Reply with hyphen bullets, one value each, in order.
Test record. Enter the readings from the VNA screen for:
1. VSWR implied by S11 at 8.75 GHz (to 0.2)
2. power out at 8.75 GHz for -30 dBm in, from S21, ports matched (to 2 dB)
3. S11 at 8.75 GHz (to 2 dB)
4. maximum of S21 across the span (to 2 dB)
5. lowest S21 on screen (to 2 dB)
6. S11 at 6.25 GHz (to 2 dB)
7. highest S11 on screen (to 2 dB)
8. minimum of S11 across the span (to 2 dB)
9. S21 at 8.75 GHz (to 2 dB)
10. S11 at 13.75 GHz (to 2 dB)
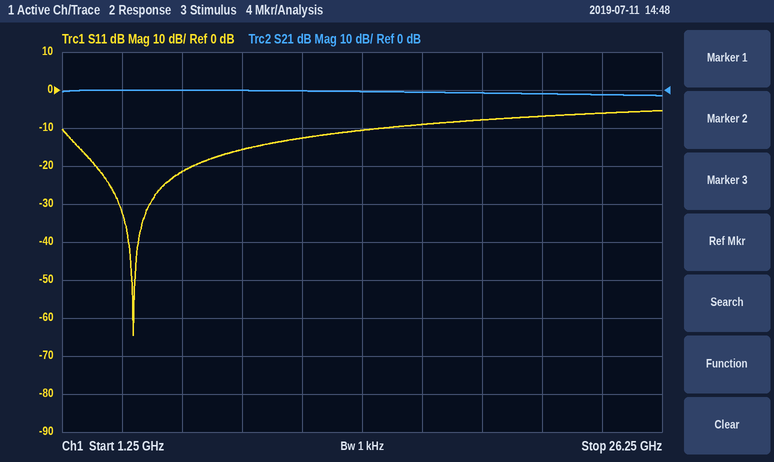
- 1.4
- -30 dBm
- -16 dB
- 0 dB
- -2 dB
- -22 dB
- -6 dB
- -64 dB
- 0 dB
- -10 dB
